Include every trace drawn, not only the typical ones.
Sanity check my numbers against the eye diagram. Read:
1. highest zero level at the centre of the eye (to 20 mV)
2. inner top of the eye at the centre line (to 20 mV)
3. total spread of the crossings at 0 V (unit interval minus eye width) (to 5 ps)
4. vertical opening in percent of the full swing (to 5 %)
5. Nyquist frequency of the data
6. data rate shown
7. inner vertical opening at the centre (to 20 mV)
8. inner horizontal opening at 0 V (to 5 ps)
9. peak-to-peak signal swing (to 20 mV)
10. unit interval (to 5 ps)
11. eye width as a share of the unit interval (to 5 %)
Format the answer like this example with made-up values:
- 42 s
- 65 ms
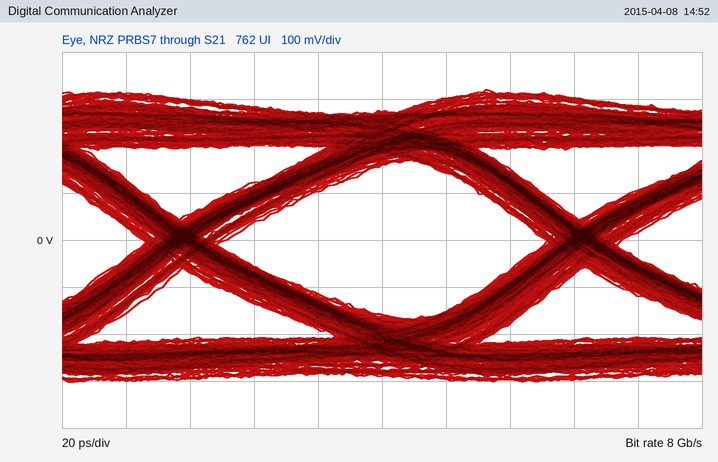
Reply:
- -160 mV
- 160 mV
- 25 ps
- 50 %
- 4 GHz
- 8 Gb/s
- 320 mV
- 100 ps
- 620 mV
- 125 ps
- 80 %
